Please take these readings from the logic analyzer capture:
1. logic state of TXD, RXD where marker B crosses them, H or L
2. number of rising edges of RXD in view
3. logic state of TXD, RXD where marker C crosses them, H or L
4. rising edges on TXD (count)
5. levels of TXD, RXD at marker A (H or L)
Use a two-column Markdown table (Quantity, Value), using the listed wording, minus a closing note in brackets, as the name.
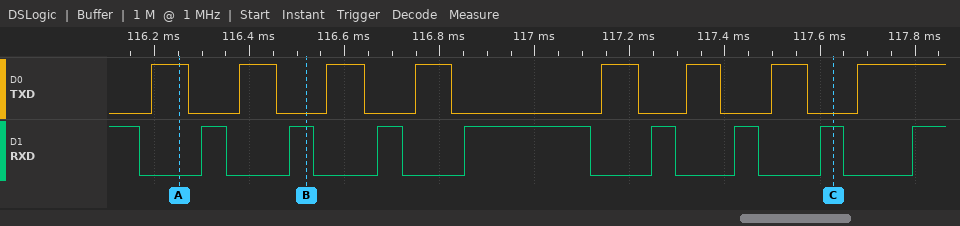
| Quantity | Value |
|---|---|
| logic state of TXD, RXD where marker B crosses them, H or L | TXD=L, RXD=H |
| number of rising edges of RXD in view | 8 |
| logic state of TXD, RXD where marker C crosses them, H or L | TXD=L, RXD=H |
| rising edges on TXD | 8 |
| levels of TXD, RXD at marker A | TXD=H, RXD=L |
